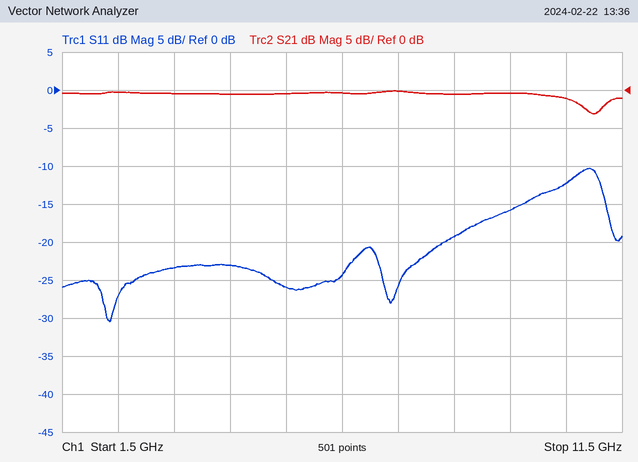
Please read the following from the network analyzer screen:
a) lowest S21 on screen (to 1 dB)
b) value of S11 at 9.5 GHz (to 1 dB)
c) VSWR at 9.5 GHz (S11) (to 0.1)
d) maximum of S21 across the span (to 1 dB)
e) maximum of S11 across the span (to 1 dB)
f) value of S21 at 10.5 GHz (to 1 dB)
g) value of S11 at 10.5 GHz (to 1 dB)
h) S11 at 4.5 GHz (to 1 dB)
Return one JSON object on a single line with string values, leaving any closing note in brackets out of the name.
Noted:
{"lowest S21 on screen": "-3 dB", "value of S11 at 9.5 GHz": "-16 dB", "VSWR at 9.5 GHz (S11)": "1.4", "maximum of S21 across the span": "0 dB", "maximum of S11 across the span": "-10 dB", "value of S21 at 10.5 GHz": "-1 dB", "value of S11 at 10.5 GHz": "-12 dB", "S11 at 4.5 GHz": "-23 dB"}
